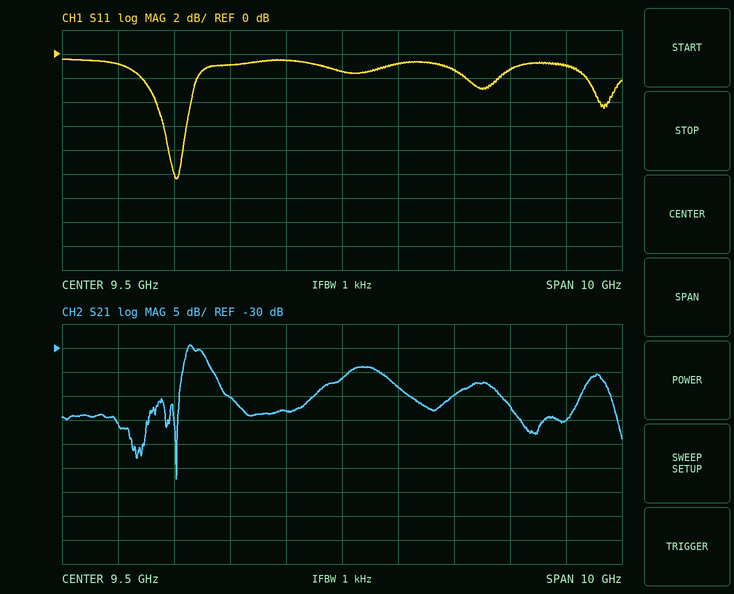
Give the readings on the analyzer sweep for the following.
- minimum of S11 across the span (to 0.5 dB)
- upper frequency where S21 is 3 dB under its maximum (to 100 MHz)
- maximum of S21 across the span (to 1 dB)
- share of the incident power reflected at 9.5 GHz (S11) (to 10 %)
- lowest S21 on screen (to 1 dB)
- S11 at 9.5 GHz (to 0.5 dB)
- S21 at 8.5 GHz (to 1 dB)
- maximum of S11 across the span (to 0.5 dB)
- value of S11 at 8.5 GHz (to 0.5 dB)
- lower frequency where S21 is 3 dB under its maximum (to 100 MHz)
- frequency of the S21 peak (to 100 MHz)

-10.5 dB
7.1 GHz
-29 dB
70 %
-57 dB
-1.5 dB
-43 dB
-0.5 dB
-0.5 dB
6.7 GHz
6.8 GHz
